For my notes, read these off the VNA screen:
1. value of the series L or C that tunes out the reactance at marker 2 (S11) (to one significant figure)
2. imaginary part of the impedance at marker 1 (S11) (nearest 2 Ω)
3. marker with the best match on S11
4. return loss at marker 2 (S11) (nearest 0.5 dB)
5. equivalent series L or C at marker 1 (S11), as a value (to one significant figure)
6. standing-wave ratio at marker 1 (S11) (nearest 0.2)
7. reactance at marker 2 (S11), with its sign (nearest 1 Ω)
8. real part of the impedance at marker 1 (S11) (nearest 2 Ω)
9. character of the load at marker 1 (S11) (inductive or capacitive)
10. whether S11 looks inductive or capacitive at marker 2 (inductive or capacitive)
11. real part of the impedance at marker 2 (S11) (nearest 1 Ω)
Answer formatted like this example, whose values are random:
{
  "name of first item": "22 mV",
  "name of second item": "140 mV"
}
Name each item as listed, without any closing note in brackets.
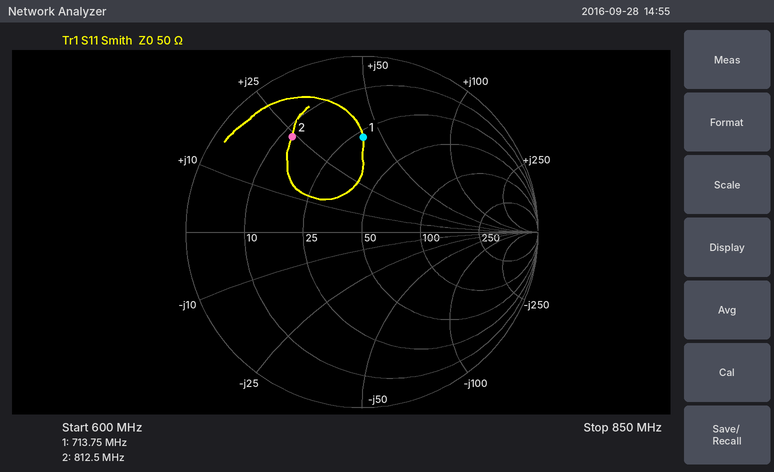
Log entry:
{
  "value of the series L or C that tunes out the reactance at marker 2 (S11)": "8 pF",
  "imaginary part of the impedance at marker 1 (S11)": "+42 Ω",
  "marker with the best match on S11": "marker 1",
  "return loss at marker 2 (S11)": "3.5 dB",
  "equivalent series L or C at marker 1 (S11), as a value": "9 nH",
  "standing-wave ratio at marker 1 (S11)": "3.4",
  "reactance at marker 2 (S11), with its sign": "+24 Ω",
  "real part of the impedance at marker 1 (S11)": "28 Ω",
  "character of the load at marker 1 (S11)": "inductive",
  "whether S11 looks inductive or capacitive at marker 2": "inductive",
  "real part of the impedance at marker 2 (S11)": "12 Ω"
}
